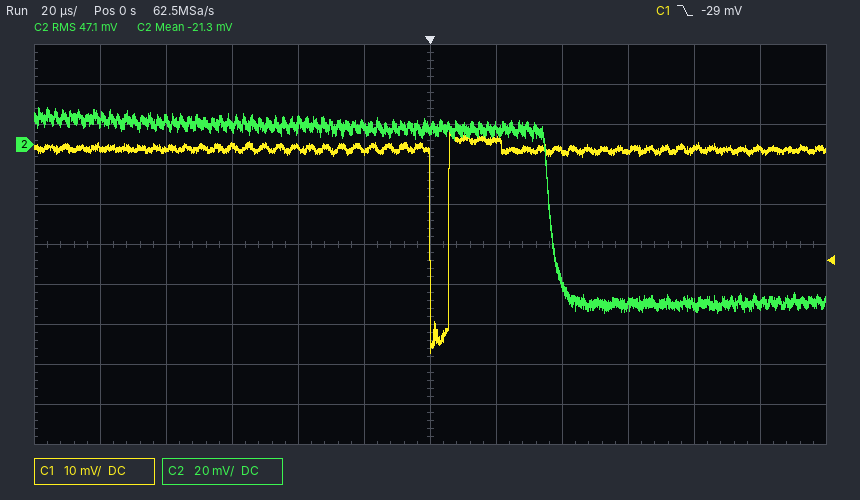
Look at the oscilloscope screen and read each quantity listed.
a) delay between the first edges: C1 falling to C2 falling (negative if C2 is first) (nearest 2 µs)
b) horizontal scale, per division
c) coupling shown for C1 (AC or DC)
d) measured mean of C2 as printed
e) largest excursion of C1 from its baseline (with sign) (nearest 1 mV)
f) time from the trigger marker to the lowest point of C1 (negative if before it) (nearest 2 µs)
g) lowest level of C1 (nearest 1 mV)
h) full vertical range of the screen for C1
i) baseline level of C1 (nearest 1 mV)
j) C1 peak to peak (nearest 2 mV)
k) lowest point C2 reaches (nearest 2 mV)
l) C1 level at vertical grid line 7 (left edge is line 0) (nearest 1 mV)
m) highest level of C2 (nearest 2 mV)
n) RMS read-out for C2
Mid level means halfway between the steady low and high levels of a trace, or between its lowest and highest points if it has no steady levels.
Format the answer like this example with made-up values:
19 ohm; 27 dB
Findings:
+36 µs; 20 µs; DC; -21.3 mV; -51 mV; 0 µs; -52 mV; 100 mV; -1 mV; 56 mV; -84 mV; 1 mV; 18 mV; 47.1 mV
